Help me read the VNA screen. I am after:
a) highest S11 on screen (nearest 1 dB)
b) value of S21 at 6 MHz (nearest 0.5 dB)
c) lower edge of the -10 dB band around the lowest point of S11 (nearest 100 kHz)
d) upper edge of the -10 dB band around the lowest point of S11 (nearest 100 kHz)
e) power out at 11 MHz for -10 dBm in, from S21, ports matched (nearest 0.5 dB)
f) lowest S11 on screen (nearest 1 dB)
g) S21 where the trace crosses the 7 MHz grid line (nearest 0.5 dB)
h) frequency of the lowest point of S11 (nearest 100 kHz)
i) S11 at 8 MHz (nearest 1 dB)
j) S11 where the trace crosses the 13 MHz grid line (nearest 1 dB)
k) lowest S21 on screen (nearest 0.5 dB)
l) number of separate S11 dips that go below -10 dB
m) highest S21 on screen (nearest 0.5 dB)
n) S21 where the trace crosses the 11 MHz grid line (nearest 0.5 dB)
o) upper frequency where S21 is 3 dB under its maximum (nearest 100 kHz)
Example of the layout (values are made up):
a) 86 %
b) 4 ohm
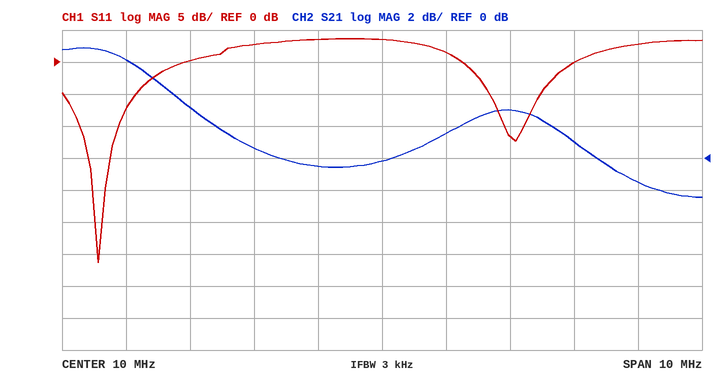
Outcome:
a) 4 dB
b) 6.0 dB
c) 5.3 MHz
d) 5.9 MHz
e) -8.5 dBm
f) -31 dB
g) 3.0 dB
h) 5.6 MHz
i) 3 dB
j) 0 dB
k) -2.5 dB
l) 2
m) 7.0 dB
n) 1.5 dB
o) 6.8 MHz
